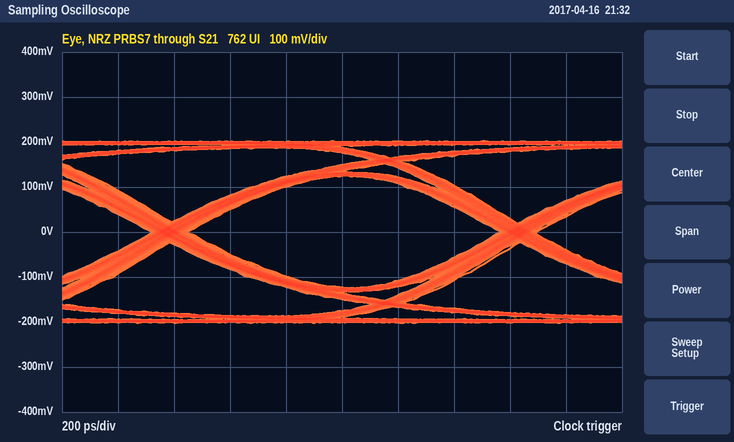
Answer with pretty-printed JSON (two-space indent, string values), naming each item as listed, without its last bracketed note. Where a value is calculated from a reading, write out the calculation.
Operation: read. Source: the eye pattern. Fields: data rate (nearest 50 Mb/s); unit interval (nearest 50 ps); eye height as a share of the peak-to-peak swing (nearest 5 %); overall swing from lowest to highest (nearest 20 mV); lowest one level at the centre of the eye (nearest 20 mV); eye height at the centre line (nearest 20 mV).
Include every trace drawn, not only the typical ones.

{
  "data rate": "800 Mb/s",
  "unit interval": "1.25 ns",
  "eye height as a share of the peak-to-peak swing": "240 mV / 400 mV ≈ 60 %",
  "overall swing from lowest to highest": "400 mV",
  "lowest one level at the centre of the eye": "120 mV",
  "eye height at the centre line": "240 mV"
}
